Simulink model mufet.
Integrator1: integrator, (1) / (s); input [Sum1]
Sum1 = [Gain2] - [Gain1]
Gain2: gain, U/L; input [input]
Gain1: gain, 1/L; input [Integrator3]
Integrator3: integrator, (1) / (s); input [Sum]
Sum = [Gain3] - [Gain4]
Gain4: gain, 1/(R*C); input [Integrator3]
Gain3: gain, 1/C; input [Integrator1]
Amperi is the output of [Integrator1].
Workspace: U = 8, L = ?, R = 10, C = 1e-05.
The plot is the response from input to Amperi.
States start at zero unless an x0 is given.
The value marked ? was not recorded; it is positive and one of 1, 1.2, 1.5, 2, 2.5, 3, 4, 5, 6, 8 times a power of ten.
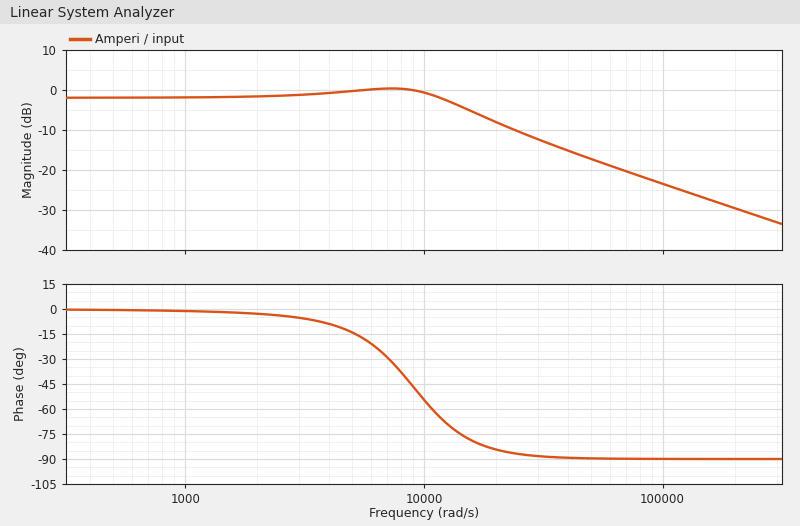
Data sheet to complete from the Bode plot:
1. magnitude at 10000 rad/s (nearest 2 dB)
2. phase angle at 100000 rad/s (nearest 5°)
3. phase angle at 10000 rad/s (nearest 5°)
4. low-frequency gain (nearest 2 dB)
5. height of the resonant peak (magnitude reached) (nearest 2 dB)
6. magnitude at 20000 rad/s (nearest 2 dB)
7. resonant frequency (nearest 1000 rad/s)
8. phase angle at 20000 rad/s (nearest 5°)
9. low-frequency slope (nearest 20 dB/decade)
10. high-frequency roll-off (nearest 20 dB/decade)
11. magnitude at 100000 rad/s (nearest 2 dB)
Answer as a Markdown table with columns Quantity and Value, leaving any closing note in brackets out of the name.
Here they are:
| Quantity | Value |
|---|---|
| magnitude at 10000 rad/s | 0 dB |
| phase angle at 100000 rad/s | -90° |
| phase angle at 10000 rad/s | -55° |
| low-frequency gain | -2 dB |
| height of the resonant peak (magnitude reached) | 0 dB |
| magnitude at 20000 rad/s | -8 dB |
| resonant frequency | 7000 rad/s |
| phase angle at 20000 rad/s | -85° |
| low-frequency slope | 0 dB/decade |
| high-frequency roll-off | -20 dB/decade |
| magnitude at 100000 rad/s | -24 dB |
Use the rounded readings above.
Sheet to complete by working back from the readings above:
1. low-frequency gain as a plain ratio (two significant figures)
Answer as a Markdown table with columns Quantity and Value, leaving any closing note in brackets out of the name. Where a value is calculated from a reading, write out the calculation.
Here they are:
| Quantity | Value |
|---|---|
| low-frequency gain as a plain ratio | 10^(-2 / 20) = 0.79 |
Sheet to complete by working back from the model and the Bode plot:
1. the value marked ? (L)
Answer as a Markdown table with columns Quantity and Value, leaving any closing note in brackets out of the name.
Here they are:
| Quantity | Value |
|---|---|
| the value marked ? | 0.0012 |
